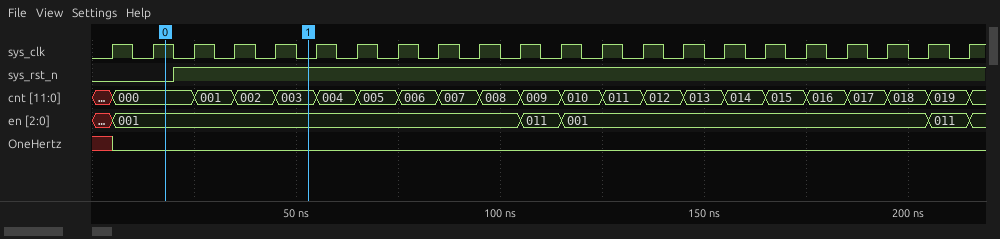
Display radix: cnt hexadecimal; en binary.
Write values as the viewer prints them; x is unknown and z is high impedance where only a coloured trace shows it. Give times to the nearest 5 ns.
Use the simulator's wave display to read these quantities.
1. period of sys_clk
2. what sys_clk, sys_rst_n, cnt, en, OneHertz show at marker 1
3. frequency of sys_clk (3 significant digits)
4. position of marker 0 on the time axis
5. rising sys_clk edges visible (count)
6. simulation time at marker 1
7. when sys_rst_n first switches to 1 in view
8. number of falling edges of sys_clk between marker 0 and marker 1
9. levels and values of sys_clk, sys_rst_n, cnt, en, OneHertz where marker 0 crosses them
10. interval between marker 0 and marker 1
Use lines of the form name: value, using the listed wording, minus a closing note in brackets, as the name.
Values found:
period of sys_clk: 10 ns
what sys_clk, sys_rst_n, cnt, en, OneHertz show at marker 1: sys_clk=0, sys_rst_n=1, cnt=003, en=001, OneHertz=0
frequency of sys_clk: 100 MHz
position of marker 0 on the time axis: 20 ns
rising sys_clk edges visible: 22
simulation time at marker 1: 55 ns
when sys_rst_n first switches to 1 in view: 20 ns
number of falling edges of sys_clk between marker 0 and marker 1: 4
levels and values of sys_clk, sys_rst_n, cnt, en, OneHertz where marker 0 crosses them: sys_clk=1, sys_rst_n=0, cnt=000, en=001, OneHertz=0
interval between marker 0 and marker 1: 35 ns
